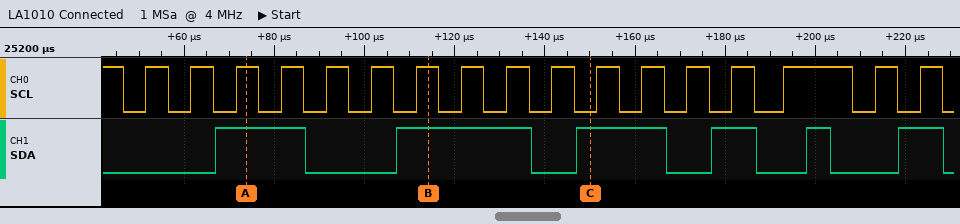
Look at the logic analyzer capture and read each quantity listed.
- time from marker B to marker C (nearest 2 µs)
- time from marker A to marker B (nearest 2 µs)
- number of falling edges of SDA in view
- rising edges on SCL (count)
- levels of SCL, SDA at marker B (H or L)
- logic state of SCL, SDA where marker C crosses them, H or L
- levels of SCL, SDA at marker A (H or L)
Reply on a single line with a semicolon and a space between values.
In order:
36 µs; 40 µs; 6; 17; SCL=H, SDA=H; SCL=L, SDA=H; SCL=H, SDA=H
